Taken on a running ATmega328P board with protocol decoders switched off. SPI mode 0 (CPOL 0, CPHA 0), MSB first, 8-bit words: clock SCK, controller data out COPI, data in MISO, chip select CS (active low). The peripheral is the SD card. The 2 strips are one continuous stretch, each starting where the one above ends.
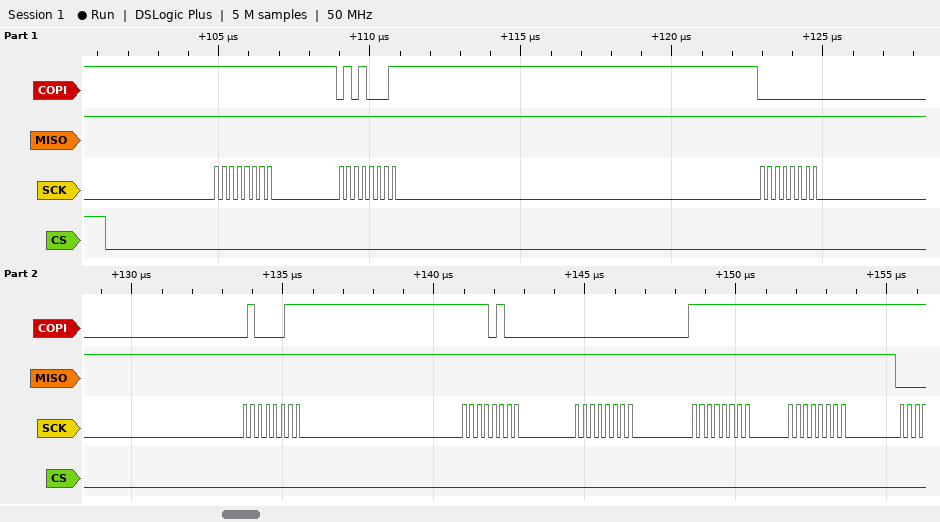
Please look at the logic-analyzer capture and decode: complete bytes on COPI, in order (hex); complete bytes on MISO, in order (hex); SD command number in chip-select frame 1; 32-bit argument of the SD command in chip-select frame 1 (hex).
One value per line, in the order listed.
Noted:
FF 51 00 43 F4 00 FF FF
FF FF FF FF FF FF FF FF
CMD17
0x0043F400
